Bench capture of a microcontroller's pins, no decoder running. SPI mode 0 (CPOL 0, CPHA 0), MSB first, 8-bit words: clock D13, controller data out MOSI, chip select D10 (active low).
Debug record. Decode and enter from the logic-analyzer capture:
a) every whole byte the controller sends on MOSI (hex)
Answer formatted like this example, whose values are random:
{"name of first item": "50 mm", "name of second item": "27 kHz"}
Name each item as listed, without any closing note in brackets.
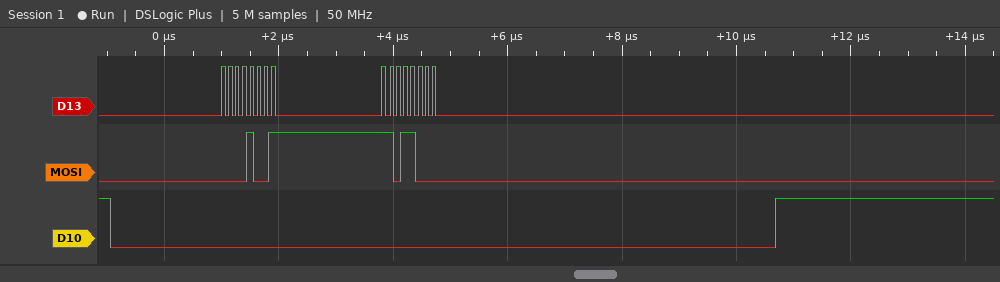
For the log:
{"every whole byte the controller sends on MOSI": "0x09 0xD8"}
